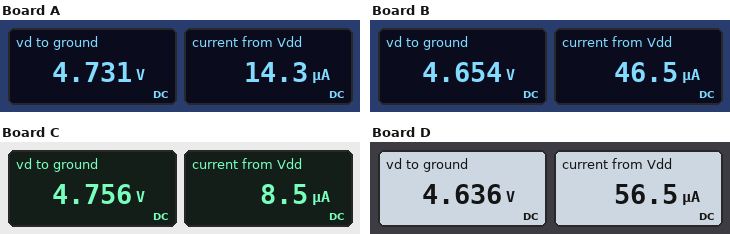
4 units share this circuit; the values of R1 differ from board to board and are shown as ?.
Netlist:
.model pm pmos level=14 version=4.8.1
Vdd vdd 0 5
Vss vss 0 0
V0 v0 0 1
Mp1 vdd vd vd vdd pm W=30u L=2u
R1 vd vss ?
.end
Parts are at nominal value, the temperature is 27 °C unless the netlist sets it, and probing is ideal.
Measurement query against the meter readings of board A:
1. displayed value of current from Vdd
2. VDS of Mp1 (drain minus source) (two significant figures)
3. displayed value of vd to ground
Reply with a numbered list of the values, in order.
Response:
1. 14.3 µA
2. 270 mV
3. 4.731 V
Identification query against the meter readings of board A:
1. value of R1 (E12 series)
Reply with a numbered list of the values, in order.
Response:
1. 330 kΩ
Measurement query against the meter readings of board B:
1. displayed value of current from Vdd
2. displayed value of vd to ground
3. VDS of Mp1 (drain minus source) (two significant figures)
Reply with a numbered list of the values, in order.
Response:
1. 46.5 µA
2. 4.654 V
3. 350 mV
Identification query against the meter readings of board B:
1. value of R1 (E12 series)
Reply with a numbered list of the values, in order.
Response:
1. 100 kΩ
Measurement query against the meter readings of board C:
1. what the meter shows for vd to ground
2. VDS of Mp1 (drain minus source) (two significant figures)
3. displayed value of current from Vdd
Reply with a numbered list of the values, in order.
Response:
1. 4.756 V
2. 240 mV
3. 8.5 µA
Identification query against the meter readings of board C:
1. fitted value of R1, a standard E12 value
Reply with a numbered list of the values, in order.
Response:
1. 560 kΩ
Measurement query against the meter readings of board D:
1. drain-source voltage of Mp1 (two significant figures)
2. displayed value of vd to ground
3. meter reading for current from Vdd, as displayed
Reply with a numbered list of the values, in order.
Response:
1. 360 mV
2. 4.636 V
3. 56.5 µA
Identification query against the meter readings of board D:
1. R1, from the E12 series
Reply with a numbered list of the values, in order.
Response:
1. 82 kΩ
